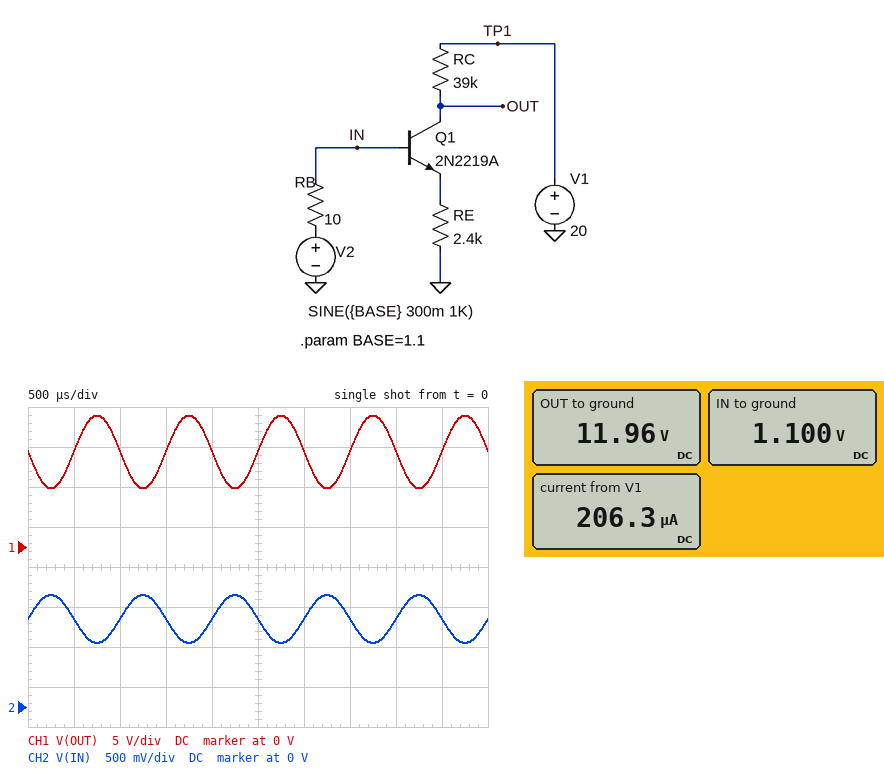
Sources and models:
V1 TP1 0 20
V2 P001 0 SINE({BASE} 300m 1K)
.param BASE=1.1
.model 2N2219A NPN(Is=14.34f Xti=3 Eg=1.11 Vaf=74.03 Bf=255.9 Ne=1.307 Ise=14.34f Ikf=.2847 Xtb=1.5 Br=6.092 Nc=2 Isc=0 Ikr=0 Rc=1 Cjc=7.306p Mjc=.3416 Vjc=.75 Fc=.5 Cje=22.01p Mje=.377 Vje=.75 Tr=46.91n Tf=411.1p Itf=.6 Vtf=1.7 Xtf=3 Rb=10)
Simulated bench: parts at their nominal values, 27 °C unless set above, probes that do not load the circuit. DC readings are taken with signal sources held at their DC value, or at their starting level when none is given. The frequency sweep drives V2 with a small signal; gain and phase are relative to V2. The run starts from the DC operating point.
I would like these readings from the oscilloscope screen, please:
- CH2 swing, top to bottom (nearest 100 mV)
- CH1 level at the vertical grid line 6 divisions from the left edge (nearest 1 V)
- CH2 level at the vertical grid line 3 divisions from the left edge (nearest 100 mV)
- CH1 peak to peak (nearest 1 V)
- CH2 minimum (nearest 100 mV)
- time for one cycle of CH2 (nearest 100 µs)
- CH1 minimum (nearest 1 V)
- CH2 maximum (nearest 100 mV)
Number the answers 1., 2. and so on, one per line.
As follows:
1. 600 mV
2. 12 V
3. 1.1 V
4. 9 V
5. 800 mV
6. 1.0 ms
7. 7 V
8. 1.4 V
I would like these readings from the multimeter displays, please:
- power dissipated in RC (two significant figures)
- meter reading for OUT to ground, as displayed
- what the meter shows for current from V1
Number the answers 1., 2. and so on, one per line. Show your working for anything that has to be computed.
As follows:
1. (20 V - 11.96 V)^2 / 39 kΩ = 1.7 mW
2. 11.96 V
3. 206.3 µA
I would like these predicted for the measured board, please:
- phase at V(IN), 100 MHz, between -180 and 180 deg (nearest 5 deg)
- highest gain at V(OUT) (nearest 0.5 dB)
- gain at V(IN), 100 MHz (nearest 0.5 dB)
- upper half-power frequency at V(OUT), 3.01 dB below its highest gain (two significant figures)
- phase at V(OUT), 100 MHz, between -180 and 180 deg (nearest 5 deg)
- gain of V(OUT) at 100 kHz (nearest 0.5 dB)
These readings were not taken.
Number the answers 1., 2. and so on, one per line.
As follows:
1. 0 deg
2. 23.5 dB
3. 0 dB
4. 1.4 MHz
5. 0 deg
6. 23.5 dB
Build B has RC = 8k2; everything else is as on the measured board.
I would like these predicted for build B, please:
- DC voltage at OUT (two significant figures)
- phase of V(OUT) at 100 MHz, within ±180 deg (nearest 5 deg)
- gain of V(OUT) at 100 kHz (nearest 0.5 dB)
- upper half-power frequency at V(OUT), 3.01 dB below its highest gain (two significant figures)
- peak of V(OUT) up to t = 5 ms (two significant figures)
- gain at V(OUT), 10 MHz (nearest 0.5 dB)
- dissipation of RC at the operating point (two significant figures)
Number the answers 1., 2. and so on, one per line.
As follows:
1. 18 V
2. 5 deg
3. 10.0 dB
4. 9.6 MHz
5. 19 V
6. 7.0 dB
7. 350 µW
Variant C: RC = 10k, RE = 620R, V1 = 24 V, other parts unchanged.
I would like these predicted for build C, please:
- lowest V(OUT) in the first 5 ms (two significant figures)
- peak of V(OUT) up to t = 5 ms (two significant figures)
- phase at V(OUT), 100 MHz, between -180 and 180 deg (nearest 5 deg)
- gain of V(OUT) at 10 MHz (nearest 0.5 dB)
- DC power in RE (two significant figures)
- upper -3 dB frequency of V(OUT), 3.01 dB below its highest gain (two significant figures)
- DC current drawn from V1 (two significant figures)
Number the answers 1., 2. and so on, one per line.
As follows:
1. 12 V
2. 21 V
3. 20 deg
4. 18.0 dB
5. 350 µW
6. 6.1 MHz
7. 750 µA
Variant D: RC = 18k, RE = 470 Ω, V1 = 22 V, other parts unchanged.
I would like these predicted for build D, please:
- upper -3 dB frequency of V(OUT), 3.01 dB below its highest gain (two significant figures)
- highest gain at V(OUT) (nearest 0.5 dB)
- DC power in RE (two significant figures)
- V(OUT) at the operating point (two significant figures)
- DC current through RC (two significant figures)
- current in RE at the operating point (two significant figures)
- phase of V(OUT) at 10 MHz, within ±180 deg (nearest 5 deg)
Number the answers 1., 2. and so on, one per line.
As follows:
1. 2.1 MHz
2. 31.0 dB
3. 440 µW
4. 4.6 V
5. 960 µA
6. 970 µA
7. 90 deg
